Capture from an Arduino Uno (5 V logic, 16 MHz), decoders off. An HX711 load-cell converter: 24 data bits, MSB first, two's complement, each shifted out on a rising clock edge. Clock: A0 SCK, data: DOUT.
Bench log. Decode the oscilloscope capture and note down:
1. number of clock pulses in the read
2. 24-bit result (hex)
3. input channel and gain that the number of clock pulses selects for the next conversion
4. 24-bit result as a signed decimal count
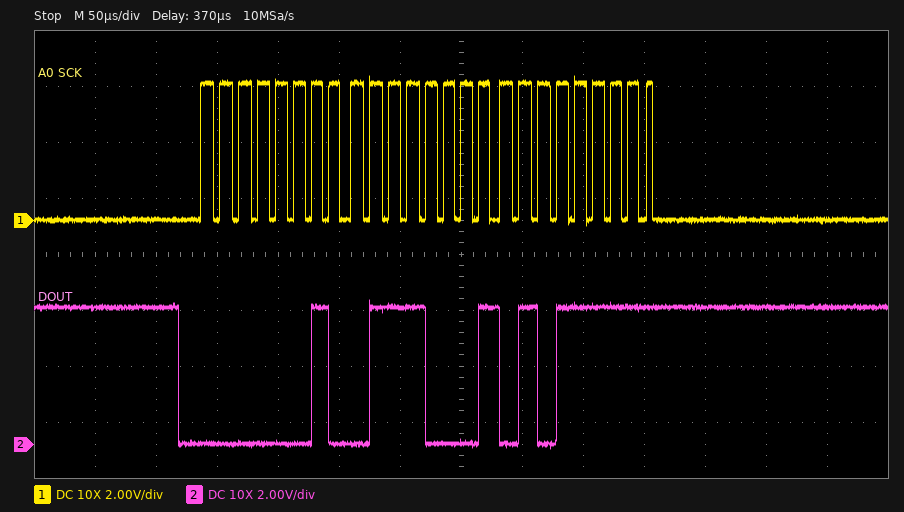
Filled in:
25
0x02715F
channel A, gain 128
160095
